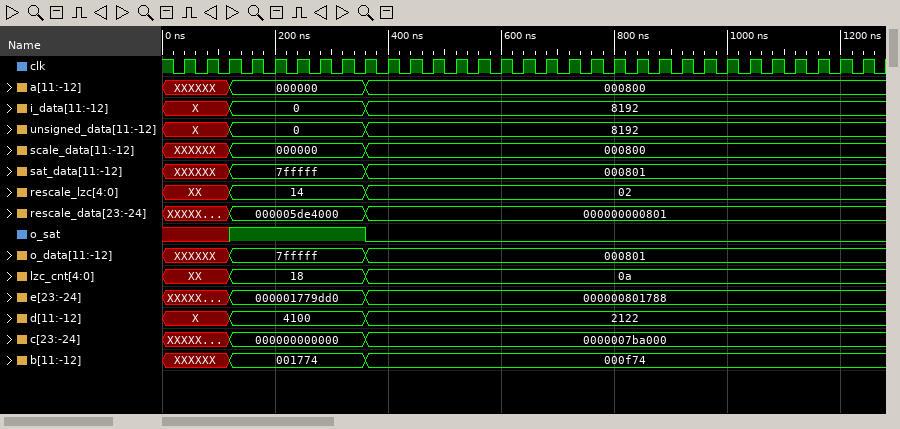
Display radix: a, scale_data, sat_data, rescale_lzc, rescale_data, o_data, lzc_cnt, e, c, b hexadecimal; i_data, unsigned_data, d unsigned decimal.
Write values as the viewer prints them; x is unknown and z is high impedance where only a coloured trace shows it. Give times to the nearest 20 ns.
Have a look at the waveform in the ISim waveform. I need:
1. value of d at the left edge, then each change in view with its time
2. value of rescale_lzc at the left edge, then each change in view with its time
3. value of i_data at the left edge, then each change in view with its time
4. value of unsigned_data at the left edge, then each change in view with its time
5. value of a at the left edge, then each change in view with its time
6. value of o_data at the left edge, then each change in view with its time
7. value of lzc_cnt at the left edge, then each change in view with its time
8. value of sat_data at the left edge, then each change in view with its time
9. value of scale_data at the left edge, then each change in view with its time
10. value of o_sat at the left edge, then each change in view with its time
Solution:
X, 4100 at 120 ns, 2122 at 360 ns
XX, 14 at 120 ns, 02 at 360 ns
X, 0 at 120 ns, 8192 at 360 ns
X, 0 at 120 ns, 8192 at 360 ns
XXXXXX, 000000 at 120 ns, 000800 at 360 ns
XXXXXX, 7fffff at 120 ns, 000801 at 360 ns
XX, 18 at 120 ns, 0a at 360 ns
XXXXXX, 7fffff at 120 ns, 000801 at 360 ns
XXXXXX, 000000 at 120 ns, 000800 at 360 ns
x, 1 at 120 ns, 0 at 360 ns
